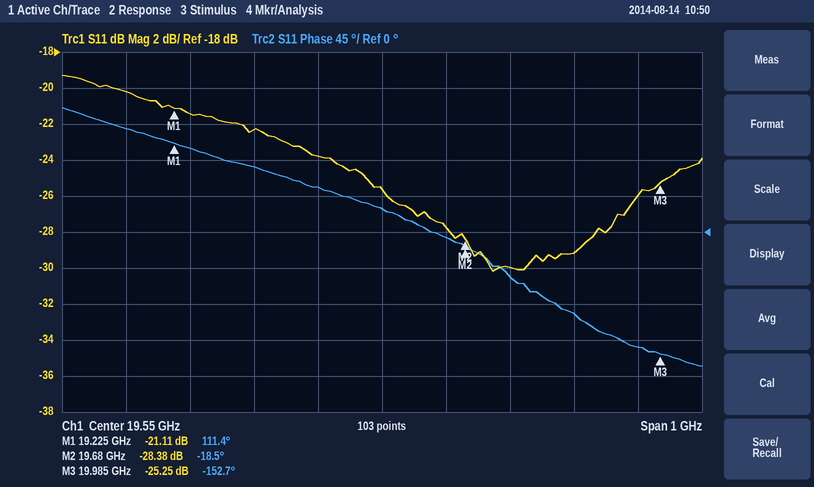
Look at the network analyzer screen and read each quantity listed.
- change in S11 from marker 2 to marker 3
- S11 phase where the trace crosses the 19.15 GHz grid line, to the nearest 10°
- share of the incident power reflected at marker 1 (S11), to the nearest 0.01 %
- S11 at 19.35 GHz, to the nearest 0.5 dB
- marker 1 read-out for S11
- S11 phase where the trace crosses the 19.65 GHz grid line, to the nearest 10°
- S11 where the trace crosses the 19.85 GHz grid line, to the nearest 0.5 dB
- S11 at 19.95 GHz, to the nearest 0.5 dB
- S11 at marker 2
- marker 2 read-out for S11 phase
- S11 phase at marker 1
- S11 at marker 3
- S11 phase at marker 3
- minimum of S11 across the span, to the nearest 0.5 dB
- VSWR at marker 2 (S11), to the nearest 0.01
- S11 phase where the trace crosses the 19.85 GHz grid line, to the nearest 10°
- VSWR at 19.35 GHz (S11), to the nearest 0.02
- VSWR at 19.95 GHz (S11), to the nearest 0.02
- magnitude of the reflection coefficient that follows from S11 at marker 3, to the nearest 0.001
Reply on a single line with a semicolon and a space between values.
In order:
3.13 dB; 130°; 0.77 %; -22.5 dB; -21.11 dB; -10°; -29.0 dB; -26.0 dB; -28.38 dB; -18.5°; 111.4°; -25.25 dB; -152.7°; -30.0 dB; 1.08; -100°; 1.16; 1.10; 0.055
